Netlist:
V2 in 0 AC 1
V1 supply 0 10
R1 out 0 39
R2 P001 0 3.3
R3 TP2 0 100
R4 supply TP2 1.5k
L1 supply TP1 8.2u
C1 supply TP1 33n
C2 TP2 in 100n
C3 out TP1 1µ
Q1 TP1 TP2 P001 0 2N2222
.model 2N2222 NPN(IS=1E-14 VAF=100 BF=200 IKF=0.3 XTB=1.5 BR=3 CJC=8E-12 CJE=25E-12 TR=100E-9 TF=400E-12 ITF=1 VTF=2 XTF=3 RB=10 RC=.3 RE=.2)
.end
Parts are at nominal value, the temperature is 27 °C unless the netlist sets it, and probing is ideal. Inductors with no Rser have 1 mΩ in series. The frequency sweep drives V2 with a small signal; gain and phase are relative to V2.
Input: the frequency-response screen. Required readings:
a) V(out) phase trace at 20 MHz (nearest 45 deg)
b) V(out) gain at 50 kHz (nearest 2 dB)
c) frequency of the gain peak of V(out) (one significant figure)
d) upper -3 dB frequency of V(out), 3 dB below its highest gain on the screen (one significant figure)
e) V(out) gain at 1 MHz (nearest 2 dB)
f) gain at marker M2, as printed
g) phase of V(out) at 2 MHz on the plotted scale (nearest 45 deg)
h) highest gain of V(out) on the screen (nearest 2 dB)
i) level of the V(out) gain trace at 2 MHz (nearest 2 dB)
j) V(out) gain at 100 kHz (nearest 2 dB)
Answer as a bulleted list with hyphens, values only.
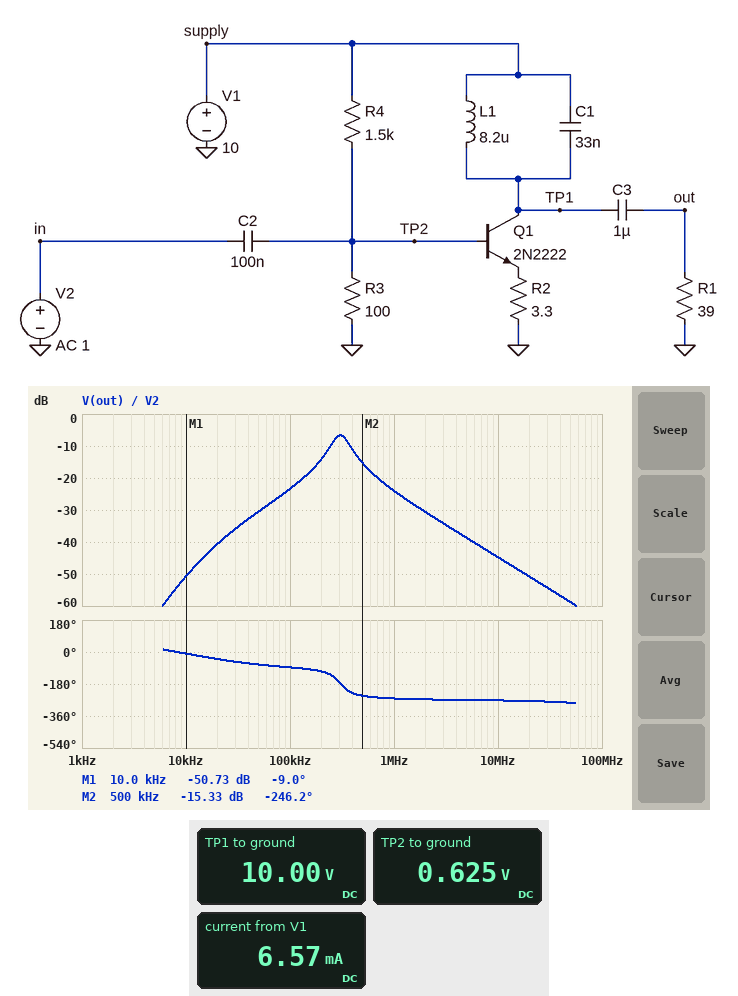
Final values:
- -270 deg
- -30 dB
- 300 kHz
- 400 kHz
- -24 dB
- -15.33 dB
- -270 deg
- -6 dB
- -30 dB
- -24 dB
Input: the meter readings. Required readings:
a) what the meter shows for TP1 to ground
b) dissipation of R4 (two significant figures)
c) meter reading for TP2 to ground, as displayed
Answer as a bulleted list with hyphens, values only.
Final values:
- 10.00 V
- 59 mW
- 0.625 V
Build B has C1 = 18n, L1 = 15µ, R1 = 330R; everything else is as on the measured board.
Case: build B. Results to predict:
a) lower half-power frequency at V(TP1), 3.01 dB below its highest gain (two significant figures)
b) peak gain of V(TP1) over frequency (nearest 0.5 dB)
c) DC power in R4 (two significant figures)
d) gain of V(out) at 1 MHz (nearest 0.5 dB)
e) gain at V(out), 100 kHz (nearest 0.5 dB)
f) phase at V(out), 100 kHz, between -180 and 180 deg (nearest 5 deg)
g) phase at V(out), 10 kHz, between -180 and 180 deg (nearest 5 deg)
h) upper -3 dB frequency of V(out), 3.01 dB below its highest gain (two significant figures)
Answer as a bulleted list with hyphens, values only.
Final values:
- 290 kHz
- 12.0 dB
- 59 mW
- -18.5 dB
- -18.0 dB
- -80 deg
- -30 deg
- 320 kHz
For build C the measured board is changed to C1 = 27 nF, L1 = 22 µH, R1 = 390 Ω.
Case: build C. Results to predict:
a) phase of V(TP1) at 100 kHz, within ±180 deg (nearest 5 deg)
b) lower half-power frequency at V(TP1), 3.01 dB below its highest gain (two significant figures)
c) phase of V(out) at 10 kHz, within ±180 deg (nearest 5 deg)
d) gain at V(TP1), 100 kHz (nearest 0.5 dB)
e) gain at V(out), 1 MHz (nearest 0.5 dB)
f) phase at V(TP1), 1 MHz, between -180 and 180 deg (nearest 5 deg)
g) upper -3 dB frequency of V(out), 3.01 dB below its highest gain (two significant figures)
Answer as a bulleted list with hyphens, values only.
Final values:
- -85 deg
- 200 kHz
- -30 deg
- -13.5 dB
- -22.5 dB
- 90 deg
- 210 kHz
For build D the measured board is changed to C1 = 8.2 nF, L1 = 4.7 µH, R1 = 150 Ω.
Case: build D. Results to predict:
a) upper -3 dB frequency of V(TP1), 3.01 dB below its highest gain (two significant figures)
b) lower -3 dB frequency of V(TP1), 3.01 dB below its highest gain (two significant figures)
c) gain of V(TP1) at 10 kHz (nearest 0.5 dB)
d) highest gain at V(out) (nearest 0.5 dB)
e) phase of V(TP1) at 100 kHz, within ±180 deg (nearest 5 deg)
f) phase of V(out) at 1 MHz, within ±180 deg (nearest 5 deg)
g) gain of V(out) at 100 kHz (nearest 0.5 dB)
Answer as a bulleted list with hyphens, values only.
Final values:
- 880 kHz
- 750 kHz
- -55.0 dB
- 5.0 dB
- -80 deg
- 110 deg
- -29.0 dB
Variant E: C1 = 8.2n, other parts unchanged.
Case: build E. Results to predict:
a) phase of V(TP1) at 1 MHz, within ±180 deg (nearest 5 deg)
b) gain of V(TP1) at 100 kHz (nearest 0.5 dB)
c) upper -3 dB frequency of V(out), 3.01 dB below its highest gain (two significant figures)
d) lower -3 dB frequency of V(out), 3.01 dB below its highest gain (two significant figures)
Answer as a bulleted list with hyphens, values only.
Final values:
- 130 deg
- -24.0 dB
- 910 kHz
- 410 kHz
